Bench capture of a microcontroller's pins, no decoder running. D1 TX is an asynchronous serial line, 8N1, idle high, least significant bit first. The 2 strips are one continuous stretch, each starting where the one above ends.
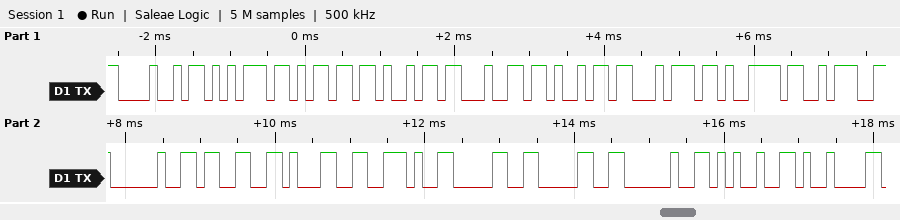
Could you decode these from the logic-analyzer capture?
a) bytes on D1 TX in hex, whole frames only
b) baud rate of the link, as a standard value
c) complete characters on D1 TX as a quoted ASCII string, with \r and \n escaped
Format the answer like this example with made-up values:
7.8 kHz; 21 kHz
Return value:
48 75 6D 69 64 69 74 79 3A 20 33 31 2E 30 30 20 25 09; 9600 baud; "Humidity: 31.00 %\t"
